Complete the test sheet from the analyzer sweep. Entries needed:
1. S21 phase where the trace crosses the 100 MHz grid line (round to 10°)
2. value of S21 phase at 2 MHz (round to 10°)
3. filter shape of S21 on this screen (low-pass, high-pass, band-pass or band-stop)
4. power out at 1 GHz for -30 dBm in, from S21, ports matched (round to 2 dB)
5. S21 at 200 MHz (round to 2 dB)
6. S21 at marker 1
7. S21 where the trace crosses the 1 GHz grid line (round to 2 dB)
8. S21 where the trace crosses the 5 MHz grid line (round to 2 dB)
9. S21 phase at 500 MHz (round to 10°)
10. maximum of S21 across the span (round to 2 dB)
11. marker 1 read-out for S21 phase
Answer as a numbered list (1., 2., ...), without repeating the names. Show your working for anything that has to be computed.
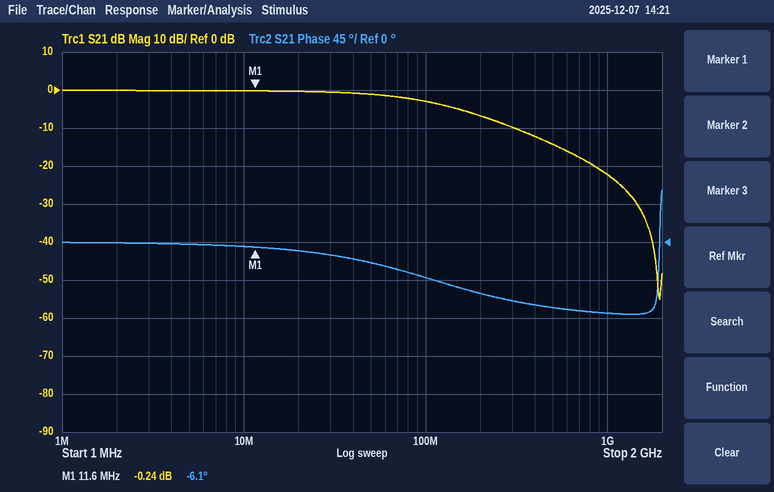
1. -40°
2. 0°
3. low-pass
4. -30 dBm + (-22 dB) = -52 dBm
5. -6 dB
6. -0.24 dB
7. -22 dB
8. 0 dB
9. -80°
10. 0 dB
11. -6.1°
